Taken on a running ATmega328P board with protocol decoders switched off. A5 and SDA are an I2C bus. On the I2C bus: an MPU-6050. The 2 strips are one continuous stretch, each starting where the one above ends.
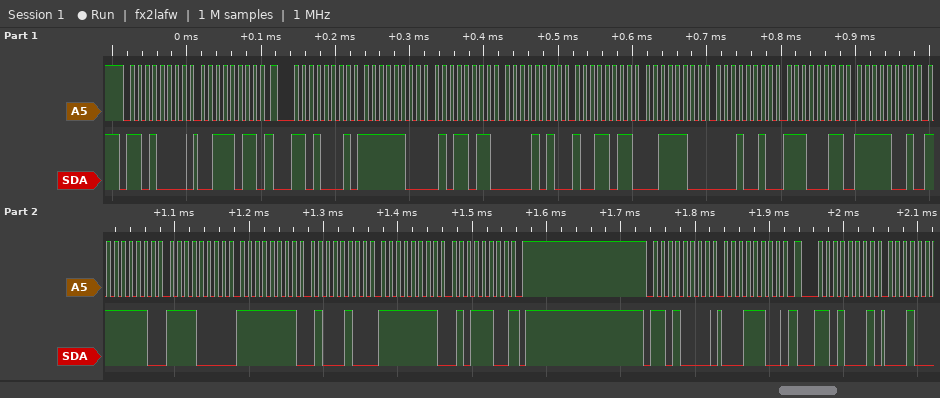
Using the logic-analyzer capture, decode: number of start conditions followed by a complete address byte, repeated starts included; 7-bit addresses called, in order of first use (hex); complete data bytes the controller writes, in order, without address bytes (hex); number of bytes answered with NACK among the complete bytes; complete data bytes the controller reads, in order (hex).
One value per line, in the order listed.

4
0x68
3B 1C
1
FC 5B 0A 9B 3C 12 E3 F9 FE F0 FF 44 FF 5C
